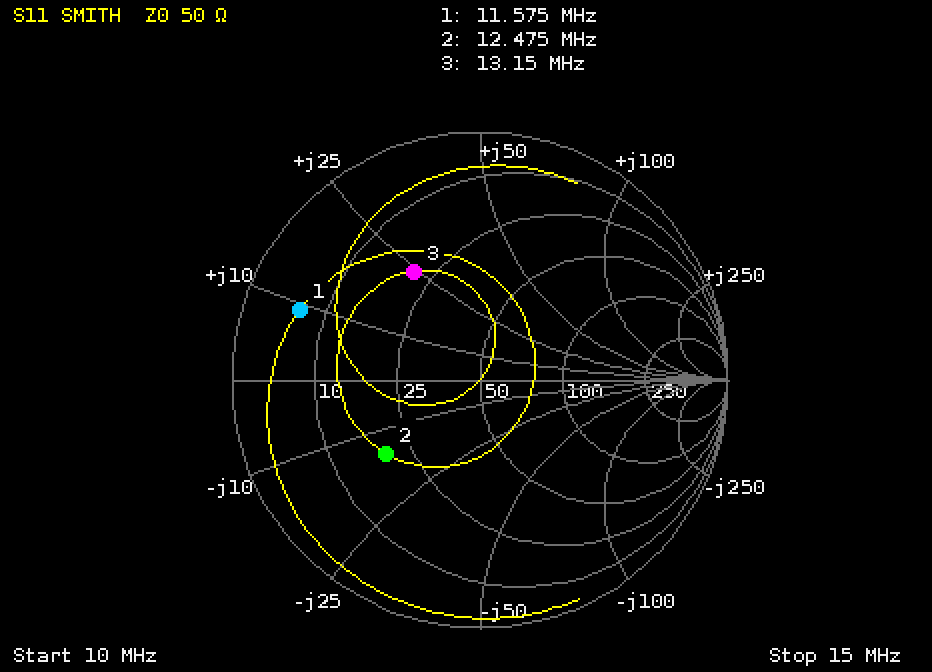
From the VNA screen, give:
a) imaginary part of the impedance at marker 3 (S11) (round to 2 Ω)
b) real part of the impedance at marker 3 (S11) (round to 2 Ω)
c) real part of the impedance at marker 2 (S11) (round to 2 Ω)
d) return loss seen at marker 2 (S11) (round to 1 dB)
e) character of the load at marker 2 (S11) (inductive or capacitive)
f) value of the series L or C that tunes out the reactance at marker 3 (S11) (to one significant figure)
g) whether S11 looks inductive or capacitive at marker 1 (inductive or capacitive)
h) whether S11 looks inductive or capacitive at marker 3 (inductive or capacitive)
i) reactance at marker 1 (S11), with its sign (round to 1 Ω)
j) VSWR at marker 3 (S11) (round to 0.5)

+24 Ω
20 Ω
20 Ω
6 dB
capacitive
500 pF
inductive
inductive
+9 Ω
3.0
